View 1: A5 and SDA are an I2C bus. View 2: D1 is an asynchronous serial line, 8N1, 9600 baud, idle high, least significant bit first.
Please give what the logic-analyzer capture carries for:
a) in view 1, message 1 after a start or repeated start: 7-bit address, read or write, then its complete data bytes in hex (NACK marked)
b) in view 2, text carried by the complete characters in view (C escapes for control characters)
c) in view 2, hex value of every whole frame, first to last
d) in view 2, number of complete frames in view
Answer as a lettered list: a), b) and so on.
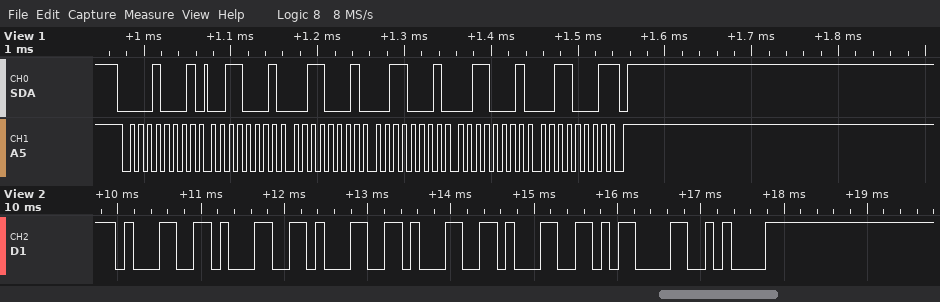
a) 0x08 read: 31 31 31 31 31 NACK
b) "11111\r\n"
c) 0x31 0x31 0x31 0x31 0x31 0x0D 0x0A
d) 7
